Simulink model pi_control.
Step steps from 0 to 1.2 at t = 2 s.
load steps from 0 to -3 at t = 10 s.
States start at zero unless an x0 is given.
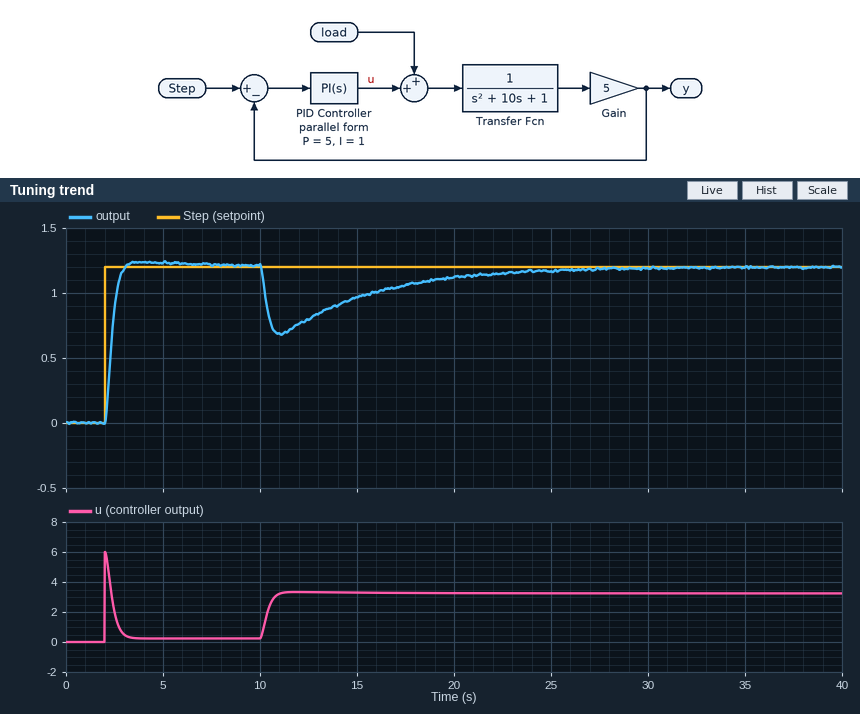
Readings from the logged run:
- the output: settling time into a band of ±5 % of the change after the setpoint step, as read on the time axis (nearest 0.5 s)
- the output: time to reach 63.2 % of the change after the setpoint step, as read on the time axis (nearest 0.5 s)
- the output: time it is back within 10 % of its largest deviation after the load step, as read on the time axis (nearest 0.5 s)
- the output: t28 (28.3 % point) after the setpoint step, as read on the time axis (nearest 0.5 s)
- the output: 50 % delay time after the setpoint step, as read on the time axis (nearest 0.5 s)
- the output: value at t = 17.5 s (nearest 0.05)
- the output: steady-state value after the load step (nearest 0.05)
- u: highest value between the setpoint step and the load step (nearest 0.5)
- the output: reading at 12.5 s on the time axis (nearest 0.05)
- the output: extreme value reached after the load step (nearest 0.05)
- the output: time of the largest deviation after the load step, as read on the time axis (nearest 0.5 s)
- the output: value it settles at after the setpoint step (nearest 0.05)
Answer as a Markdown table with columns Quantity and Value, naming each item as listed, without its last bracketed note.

| Quantity | Value |
|---|---|
| the output: settling time into a band of ±5 % of the change after the setpoint step, as read on the time axis | 3.0 s |
| the output: time to reach 63.2 % of the change after the setpoint step, as read on the time axis | 2.5 s |
| the output: time it is back within 10 % of its largest deviation after the load step, as read on the time axis | 22.0 s |
| the output: t28 (28.3 % point) after the setpoint step, as read on the time axis | 2.0 s |
| the output: 50 % delay time after the setpoint step, as read on the time axis | 2.5 s |
| the output: value at t = 17.5 s | 1.05 |
| the output: steady-state value after the load step | 1.20 |
| u: highest value between the setpoint step and the load step | 6.0 |
| the output: reading at 12.5 s on the time axis | 0.80 |
| the output: extreme value reached after the load step | 0.70 |
| the output: time of the largest deviation after the load step, as read on the time axis | 11.0 s |
| the output: value it settles at after the setpoint step | 1.20 |
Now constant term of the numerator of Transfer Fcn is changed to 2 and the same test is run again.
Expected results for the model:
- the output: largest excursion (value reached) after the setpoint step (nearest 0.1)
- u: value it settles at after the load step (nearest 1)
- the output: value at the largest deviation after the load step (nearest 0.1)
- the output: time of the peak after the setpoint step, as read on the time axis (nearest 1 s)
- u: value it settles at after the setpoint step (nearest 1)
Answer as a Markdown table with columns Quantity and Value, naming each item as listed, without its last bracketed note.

| Quantity | Value |
|---|---|
| the output: largest excursion (value reached) after the setpoint step | 1.3 |
| u: value it settles at after the load step | 3 |
| the output: value at the largest deviation after the load step | 0.6 |
| the output: time of the peak after the setpoint step, as read on the time axis | 3 s |
| u: value it settles at after the setpoint step | 0 |
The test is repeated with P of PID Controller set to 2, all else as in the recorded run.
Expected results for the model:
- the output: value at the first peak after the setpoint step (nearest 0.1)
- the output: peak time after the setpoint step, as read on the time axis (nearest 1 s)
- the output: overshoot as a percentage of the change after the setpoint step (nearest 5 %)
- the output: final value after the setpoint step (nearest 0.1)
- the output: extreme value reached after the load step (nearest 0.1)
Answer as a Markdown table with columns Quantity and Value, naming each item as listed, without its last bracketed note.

| Quantity | Value |
|---|---|
| the output: value at the first peak after the setpoint step | 1.4 |
| the output: peak time after the setpoint step, as read on the time axis | 5 s |
| the output: overshoot as a percentage of the change after the setpoint step | 15 % |
| the output: final value after the setpoint step | 1.2 |
| the output: extreme value reached after the load step | 0.2 |
